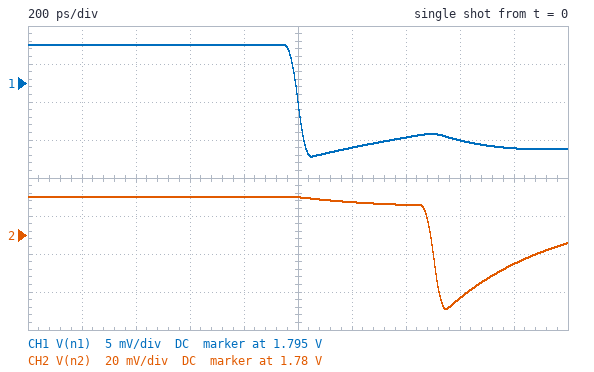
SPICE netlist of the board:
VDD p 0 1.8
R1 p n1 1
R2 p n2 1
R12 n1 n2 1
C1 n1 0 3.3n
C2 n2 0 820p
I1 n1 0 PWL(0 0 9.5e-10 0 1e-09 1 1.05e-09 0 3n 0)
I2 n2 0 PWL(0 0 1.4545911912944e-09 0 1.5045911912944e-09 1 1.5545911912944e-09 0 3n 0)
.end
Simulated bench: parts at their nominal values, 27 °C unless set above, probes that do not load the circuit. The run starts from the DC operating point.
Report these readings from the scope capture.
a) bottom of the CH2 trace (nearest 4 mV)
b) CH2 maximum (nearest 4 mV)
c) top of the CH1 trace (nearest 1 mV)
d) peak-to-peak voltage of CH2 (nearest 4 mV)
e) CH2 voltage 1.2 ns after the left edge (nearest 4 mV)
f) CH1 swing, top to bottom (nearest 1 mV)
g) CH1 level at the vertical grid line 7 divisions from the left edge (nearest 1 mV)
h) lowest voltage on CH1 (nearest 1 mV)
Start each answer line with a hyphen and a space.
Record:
- 1.740 V
- 1.800 V
- 1.800 V
- 60 mV
- 1.796 V
- 15 mV
- 1.788 V
- 1.785 V
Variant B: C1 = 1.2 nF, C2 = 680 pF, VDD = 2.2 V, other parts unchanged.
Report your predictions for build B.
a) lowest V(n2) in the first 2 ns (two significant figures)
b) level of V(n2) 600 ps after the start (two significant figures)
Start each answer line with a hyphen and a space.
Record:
- 2.1 V
- 2.2 V
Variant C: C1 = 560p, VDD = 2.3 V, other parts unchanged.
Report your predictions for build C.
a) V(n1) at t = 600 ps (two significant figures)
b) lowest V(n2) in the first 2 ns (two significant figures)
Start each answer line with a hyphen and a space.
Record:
- 2.3 V
- 2.2 V
